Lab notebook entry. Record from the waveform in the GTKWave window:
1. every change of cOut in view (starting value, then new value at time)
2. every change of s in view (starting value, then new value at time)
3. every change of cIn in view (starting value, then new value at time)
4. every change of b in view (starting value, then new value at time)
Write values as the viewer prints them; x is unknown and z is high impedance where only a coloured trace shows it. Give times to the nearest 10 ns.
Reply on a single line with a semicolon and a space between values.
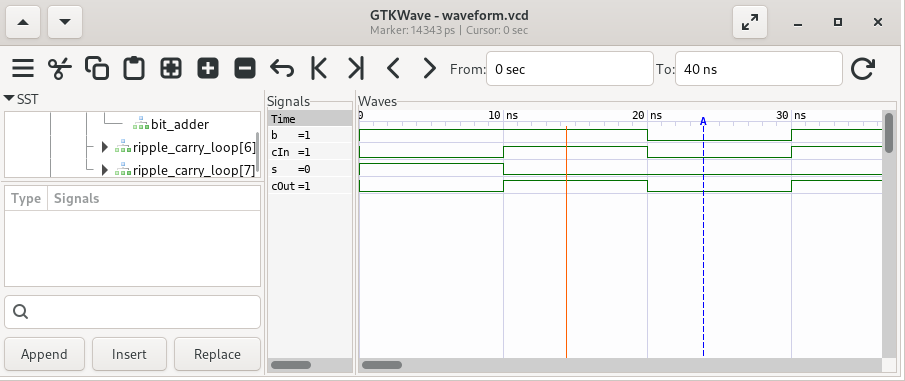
0, 1 at 10 ns, 0 at 20 ns, 1 at 30 ns; 1, 0 at 10 ns; 0, 1 at 10 ns, 0 at 20 ns, 1 at 30 ns; 1, 0 at 20 ns, 1 at 30 ns
